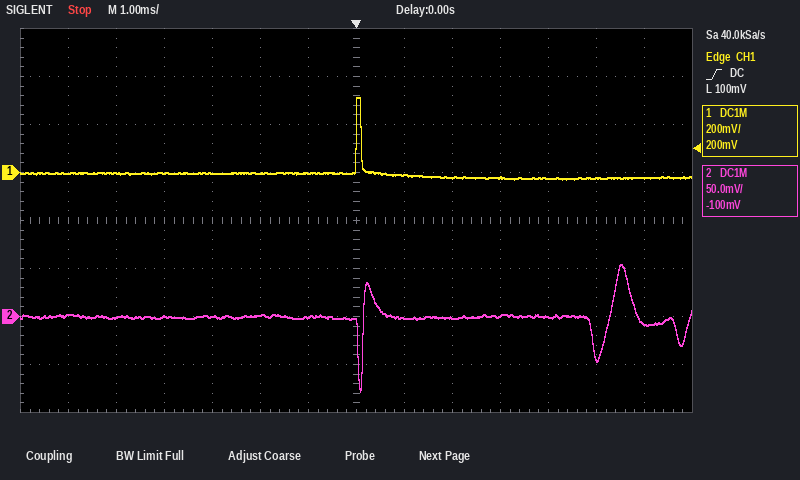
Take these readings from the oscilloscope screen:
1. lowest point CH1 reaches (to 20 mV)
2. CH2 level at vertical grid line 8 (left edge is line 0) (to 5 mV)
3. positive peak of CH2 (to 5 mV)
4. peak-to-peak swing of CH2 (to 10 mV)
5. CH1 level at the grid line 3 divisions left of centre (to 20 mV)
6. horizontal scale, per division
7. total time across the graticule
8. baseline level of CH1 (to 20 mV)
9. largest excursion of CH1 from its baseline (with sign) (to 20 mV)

-20 mV
0 mV
55 mV
130 mV
0 mV
1 ms
14 ms
0 mV
+320 mV
